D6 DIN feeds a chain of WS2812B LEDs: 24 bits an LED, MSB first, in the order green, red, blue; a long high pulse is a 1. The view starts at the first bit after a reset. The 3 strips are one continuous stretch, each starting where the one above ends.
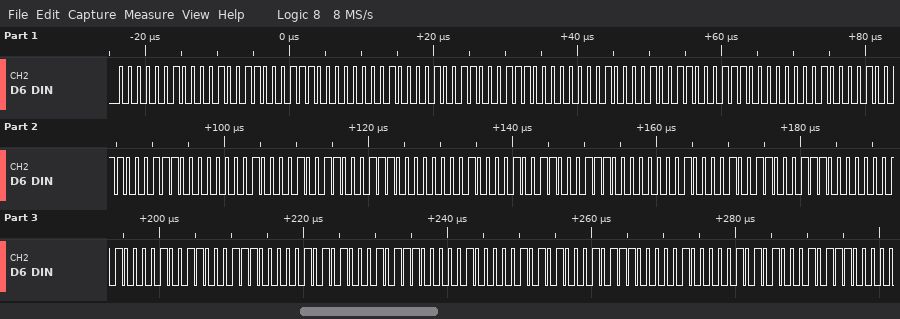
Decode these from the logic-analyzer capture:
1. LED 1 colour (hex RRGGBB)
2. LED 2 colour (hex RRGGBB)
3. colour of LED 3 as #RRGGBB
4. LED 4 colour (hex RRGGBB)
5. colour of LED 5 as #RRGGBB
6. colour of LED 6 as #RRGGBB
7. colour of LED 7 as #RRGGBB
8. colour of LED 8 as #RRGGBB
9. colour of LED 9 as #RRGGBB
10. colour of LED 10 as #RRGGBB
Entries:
#13021C
#13021C
#13021C
#13021C
#13021C
#13021C
#13021C
#13021C
#171504
#171504
